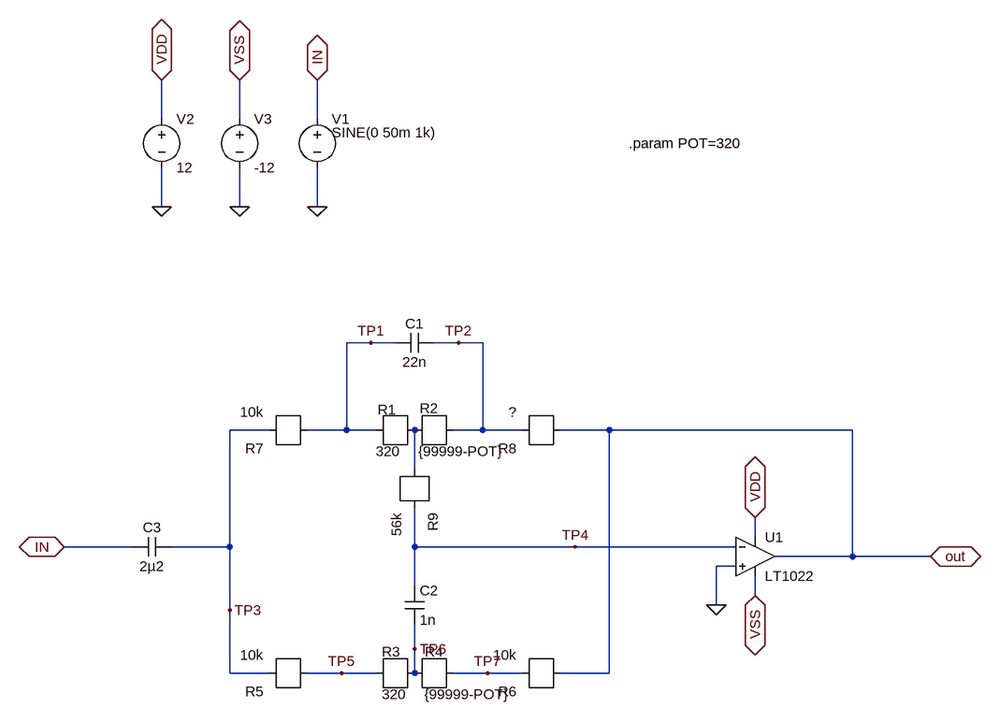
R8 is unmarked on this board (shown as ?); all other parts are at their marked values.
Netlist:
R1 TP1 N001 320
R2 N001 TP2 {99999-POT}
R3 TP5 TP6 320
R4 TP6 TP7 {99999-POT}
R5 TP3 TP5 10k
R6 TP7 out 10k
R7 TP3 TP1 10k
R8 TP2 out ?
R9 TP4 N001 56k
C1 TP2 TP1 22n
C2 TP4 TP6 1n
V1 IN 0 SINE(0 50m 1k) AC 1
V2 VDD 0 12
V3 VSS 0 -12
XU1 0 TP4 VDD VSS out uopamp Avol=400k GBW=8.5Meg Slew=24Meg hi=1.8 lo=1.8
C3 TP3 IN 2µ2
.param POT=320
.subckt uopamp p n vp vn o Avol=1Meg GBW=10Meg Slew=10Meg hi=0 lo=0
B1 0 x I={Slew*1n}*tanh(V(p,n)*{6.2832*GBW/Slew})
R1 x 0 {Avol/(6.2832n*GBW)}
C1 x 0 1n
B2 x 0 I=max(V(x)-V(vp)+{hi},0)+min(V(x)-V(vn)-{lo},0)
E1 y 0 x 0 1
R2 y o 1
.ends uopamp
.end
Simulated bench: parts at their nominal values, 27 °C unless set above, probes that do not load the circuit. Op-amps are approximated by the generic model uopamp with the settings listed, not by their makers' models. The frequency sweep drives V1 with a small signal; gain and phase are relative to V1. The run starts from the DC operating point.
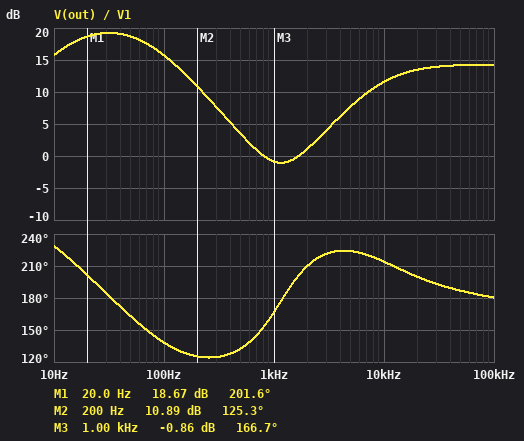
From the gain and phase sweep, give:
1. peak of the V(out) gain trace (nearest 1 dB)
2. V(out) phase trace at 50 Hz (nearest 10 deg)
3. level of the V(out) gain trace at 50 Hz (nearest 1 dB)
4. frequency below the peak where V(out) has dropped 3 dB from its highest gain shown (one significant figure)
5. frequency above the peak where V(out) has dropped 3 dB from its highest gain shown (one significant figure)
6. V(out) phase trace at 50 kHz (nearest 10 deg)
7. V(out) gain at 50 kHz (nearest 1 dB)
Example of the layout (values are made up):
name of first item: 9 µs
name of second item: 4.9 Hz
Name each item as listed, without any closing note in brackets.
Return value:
peak of the V(out) gain trace: 19 dB
V(out) phase trace at 50 Hz: 160 deg
level of the V(out) gain trace at 50 Hz: 19 dB
frequency below the peak where V(out) has dropped 3 dB from its highest gain shown: 10 Hz
frequency above the peak where V(out) has dropped 3 dB from its highest gain shown: 90 Hz
V(out) phase trace at 50 kHz: 190 deg
V(out) gain at 50 kHz: 14 dB
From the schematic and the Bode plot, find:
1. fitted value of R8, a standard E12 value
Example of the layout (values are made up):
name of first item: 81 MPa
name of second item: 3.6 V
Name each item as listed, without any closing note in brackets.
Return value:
fitted value of R8, a standard E12 value: 5.6 kΩ
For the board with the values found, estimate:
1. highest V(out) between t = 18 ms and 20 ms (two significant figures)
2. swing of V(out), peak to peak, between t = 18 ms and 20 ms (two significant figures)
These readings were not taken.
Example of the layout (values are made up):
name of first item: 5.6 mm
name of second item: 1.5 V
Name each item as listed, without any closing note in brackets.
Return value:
highest V(out) between t = 18 ms and 20 ms: 47 mV
swing of V(out), peak to peak, between t = 18 ms and 20 ms: 91 mV
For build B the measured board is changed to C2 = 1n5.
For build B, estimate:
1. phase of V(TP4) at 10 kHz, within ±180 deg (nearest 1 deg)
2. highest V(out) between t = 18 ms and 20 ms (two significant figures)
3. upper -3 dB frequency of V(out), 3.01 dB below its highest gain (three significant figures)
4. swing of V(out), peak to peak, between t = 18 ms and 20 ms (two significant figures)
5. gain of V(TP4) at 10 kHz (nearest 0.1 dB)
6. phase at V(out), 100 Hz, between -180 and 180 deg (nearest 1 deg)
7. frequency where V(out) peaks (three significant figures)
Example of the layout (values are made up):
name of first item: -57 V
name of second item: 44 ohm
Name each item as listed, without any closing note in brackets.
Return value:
phase of V(TP4) at 10 kHz, within ±180 deg: 115 deg
highest V(out) between t = 18 ms and 20 ms: 54 mV
upper -3 dB frequency of V(out), 3.01 dB below its highest gain: 90.7 Hz
swing of V(out), peak to peak, between t = 18 ms and 20 ms: 100 mV
gain of V(TP4) at 10 kHz: -45.7 dB
phase at V(out), 100 Hz, between -180 and 180 deg: 139 deg
frequency where V(out) peaks: 31.4 Hz
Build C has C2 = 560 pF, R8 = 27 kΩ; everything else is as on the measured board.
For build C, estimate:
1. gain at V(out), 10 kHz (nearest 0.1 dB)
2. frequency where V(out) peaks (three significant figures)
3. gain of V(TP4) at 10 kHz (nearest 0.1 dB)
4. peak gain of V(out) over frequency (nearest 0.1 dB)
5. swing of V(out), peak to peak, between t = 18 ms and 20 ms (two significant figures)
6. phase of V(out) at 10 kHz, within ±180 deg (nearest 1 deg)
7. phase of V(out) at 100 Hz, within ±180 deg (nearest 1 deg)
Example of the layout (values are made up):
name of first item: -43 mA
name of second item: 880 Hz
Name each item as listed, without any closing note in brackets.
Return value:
gain at V(out), 10 kHz: 15.7 dB
frequency where V(out) peaks: 33.7 Hz
gain of V(TP4) at 10 kHz: -42.9 dB
peak gain of V(out) over frequency: 20.8 dB
swing of V(out), peak to peak, between t = 18 ms and 20 ms: 290 mV
phase of V(out) at 10 kHz, within ±180 deg: -155 deg
phase of V(out) at 100 Hz, within ±180 deg: 150 deg
